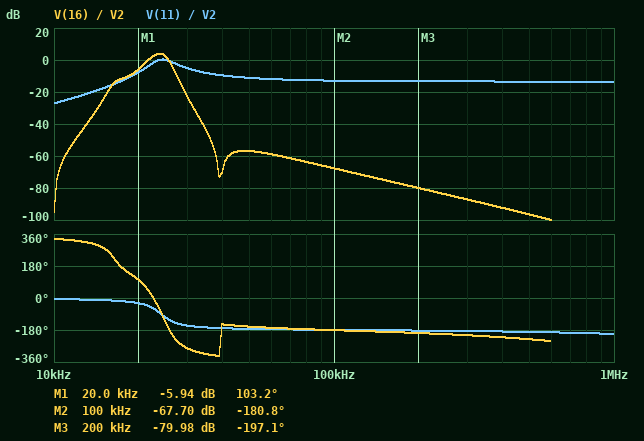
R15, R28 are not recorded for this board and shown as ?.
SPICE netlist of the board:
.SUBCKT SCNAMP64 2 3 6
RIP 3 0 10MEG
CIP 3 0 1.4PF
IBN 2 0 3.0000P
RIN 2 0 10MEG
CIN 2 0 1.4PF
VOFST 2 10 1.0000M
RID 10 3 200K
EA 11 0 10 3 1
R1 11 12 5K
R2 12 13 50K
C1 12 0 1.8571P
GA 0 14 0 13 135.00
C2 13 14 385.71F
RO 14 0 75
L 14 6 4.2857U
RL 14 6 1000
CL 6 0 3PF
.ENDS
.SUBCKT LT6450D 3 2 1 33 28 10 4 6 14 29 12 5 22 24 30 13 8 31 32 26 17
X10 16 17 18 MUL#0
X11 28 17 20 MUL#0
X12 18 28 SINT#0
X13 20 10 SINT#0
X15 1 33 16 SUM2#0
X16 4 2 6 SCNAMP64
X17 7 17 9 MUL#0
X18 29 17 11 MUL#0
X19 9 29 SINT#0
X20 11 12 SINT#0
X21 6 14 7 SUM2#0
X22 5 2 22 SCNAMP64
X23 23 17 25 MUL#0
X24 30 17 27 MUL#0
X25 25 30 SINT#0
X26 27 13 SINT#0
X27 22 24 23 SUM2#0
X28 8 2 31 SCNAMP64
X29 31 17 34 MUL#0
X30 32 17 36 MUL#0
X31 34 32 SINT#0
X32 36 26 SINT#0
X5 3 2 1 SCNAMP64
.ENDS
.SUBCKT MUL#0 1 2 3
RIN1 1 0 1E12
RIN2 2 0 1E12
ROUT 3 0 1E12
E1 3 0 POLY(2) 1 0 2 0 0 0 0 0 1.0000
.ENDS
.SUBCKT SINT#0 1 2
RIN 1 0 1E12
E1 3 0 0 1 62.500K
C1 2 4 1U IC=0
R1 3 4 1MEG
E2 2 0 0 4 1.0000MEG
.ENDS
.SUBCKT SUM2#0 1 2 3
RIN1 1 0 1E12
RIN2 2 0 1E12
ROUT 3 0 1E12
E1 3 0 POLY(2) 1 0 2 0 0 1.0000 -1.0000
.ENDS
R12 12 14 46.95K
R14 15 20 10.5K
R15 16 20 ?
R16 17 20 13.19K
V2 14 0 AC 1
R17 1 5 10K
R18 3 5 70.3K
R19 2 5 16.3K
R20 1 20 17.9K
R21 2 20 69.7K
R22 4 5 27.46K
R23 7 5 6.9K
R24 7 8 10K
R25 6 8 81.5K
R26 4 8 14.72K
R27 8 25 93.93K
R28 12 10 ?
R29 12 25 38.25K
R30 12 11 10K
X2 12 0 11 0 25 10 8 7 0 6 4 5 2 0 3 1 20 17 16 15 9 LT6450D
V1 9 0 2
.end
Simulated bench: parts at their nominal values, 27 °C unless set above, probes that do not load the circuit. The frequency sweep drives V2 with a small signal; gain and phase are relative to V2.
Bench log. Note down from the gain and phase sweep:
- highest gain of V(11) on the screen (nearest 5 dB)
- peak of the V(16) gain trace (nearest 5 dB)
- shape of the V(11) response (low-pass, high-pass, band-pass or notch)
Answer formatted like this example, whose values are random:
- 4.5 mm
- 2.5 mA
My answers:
- 0 dB
- 5 dB
- high-pass
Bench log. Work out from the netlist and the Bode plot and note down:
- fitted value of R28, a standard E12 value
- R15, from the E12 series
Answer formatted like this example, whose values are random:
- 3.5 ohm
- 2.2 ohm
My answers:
- 6.8 kΩ
- 47 kΩ
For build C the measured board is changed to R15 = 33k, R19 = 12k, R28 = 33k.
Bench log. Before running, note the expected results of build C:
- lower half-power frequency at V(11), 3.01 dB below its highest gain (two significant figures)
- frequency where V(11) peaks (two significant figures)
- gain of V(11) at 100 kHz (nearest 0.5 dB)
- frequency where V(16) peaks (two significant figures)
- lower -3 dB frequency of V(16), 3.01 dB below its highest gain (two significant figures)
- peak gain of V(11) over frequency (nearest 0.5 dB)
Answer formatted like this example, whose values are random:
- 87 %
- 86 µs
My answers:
- 9.4 kHz
- 12 kHz
- -13.5 dB
- 21 kHz
- 16 kHz
- -6.5 dB
